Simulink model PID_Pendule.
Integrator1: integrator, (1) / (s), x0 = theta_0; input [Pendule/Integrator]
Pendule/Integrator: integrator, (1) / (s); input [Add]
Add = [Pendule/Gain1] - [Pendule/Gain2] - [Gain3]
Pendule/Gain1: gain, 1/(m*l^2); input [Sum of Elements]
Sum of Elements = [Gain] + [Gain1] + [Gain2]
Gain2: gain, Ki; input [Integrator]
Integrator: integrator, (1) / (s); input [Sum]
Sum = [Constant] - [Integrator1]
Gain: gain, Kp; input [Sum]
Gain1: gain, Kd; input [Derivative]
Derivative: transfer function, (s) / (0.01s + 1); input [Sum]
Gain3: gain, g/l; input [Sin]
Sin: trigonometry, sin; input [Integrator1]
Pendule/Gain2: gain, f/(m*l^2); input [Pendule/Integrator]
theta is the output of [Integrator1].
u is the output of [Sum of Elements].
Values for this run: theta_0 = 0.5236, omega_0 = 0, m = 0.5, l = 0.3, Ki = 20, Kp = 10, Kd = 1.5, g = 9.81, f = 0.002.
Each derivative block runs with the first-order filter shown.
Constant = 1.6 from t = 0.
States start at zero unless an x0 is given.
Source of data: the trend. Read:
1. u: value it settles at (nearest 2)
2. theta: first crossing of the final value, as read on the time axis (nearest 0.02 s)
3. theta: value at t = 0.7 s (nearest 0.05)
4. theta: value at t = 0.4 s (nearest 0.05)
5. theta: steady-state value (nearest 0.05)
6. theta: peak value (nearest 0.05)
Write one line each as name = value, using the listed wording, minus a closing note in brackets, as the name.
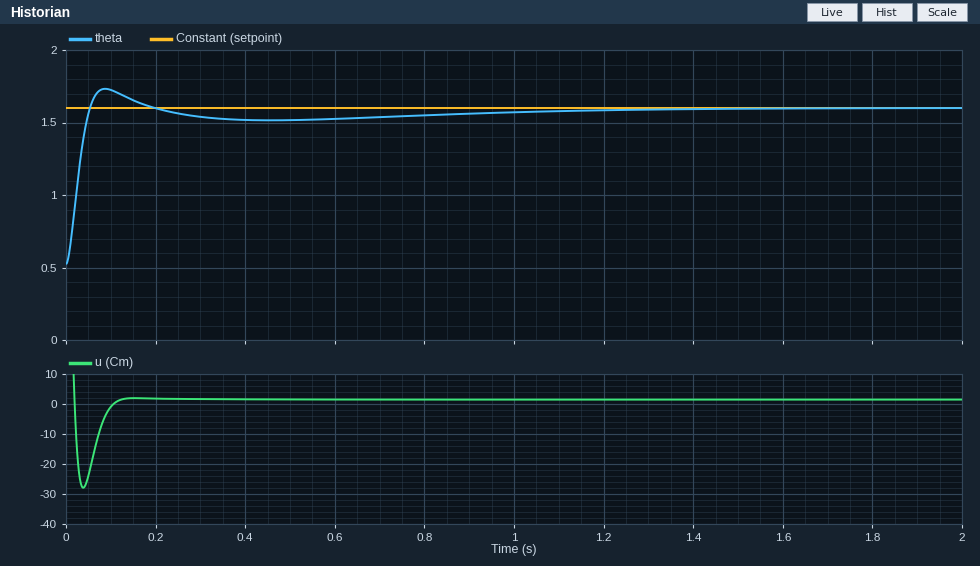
u: value it settles at = 2
theta: first crossing of the final value, as read on the time axis = 0.06 s
theta: value at t = 0.7 s = 1.55
theta: value at t = 0.4 s = 1.50
theta: steady-state value = 1.60
theta: peak value = 1.75
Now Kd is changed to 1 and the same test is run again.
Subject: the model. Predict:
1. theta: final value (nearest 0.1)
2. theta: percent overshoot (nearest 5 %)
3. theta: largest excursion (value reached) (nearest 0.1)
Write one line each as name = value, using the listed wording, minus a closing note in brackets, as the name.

theta: final value = 1.6
theta: percent overshoot = 20 %
theta: largest excursion (value reached) = 1.8
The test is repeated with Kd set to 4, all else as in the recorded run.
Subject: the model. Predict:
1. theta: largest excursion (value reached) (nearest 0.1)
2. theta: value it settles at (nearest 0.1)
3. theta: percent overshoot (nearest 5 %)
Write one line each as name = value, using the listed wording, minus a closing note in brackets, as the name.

theta: largest excursion (value reached) = 1.8
theta: value it settles at = 1.6
theta: percent overshoot = 15 %
